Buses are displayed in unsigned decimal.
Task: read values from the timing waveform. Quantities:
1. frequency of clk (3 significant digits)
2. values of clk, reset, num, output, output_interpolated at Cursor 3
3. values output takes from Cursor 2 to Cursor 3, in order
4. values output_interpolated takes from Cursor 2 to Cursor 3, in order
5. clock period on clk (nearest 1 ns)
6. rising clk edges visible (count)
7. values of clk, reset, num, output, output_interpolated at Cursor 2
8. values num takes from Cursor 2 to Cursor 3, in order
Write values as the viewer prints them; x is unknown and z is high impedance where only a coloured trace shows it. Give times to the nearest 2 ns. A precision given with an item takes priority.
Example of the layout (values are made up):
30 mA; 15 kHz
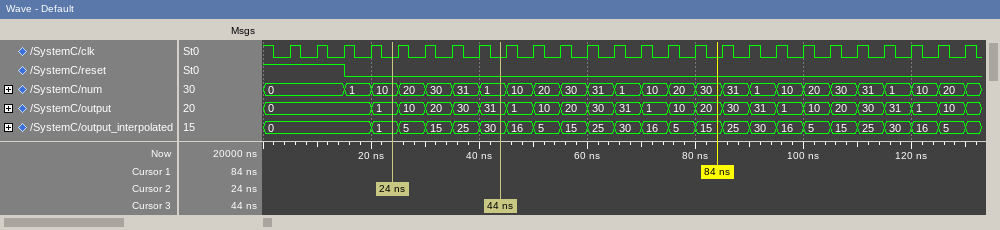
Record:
200 MHz; clk=0, reset=0, num=1, output=31, output_interpolated=30; 1, 10, 20, 30, 31; 1, 5, 15, 25, 30; 5 ns; 26; clk=0, reset=0, num=10, output=1, output_interpolated=1; 10, 20, 30, 31, 1
